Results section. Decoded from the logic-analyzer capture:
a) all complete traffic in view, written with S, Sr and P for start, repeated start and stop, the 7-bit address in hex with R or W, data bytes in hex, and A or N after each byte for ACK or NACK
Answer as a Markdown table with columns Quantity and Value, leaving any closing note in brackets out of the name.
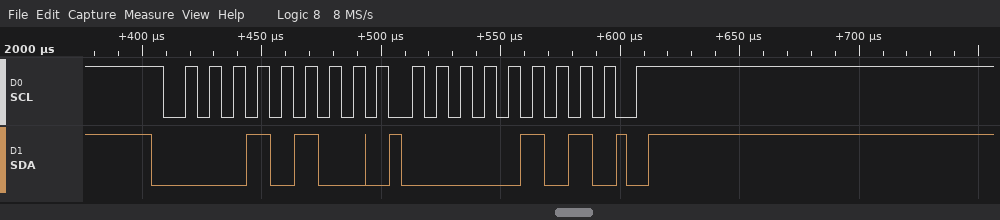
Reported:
| Quantity | Value |
|---|---|
| all complete traffic in view, written with S, Sr and P for start, repeated start and stop, the 7-bit address in hex with R or W, data bytes in hex, and A or N after each byte for ACK or NACK | S 0AW A 05 A P |
